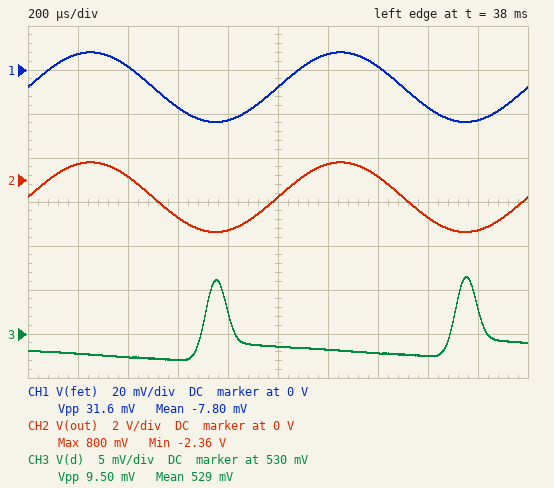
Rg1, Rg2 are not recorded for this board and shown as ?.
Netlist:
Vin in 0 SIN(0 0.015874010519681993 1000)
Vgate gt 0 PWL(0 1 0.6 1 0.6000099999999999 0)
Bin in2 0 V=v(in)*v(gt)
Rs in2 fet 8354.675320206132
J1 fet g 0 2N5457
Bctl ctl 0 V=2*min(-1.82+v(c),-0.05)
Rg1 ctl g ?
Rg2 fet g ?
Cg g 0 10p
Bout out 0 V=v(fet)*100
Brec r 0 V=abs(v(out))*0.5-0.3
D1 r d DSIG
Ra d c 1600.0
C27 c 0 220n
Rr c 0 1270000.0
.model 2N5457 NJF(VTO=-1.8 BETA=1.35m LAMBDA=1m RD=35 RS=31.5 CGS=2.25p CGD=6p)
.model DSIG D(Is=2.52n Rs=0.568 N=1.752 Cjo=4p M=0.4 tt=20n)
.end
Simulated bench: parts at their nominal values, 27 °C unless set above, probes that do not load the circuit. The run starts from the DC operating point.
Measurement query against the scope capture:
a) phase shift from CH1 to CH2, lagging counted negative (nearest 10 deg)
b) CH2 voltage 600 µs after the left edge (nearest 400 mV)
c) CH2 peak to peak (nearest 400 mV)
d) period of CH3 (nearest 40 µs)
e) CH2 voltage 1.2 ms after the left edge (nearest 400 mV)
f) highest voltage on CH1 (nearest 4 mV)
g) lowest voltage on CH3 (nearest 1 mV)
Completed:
0 deg
-1.6 V
3.2 V
1.00 ms
800 mV
8 mV
527 mV
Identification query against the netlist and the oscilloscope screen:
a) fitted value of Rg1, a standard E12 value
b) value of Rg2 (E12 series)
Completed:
560 kΩ
2.2 MΩ
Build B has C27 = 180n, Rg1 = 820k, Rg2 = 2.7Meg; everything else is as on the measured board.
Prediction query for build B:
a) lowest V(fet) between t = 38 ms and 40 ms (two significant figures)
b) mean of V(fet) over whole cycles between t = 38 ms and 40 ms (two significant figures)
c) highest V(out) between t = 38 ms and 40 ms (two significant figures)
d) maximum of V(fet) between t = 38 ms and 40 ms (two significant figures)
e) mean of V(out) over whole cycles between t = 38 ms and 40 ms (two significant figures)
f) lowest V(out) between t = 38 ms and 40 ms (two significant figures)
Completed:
-22 mV
-6.4 mV
940 mV
9.4 mV
-640 mV
-2.2 V
